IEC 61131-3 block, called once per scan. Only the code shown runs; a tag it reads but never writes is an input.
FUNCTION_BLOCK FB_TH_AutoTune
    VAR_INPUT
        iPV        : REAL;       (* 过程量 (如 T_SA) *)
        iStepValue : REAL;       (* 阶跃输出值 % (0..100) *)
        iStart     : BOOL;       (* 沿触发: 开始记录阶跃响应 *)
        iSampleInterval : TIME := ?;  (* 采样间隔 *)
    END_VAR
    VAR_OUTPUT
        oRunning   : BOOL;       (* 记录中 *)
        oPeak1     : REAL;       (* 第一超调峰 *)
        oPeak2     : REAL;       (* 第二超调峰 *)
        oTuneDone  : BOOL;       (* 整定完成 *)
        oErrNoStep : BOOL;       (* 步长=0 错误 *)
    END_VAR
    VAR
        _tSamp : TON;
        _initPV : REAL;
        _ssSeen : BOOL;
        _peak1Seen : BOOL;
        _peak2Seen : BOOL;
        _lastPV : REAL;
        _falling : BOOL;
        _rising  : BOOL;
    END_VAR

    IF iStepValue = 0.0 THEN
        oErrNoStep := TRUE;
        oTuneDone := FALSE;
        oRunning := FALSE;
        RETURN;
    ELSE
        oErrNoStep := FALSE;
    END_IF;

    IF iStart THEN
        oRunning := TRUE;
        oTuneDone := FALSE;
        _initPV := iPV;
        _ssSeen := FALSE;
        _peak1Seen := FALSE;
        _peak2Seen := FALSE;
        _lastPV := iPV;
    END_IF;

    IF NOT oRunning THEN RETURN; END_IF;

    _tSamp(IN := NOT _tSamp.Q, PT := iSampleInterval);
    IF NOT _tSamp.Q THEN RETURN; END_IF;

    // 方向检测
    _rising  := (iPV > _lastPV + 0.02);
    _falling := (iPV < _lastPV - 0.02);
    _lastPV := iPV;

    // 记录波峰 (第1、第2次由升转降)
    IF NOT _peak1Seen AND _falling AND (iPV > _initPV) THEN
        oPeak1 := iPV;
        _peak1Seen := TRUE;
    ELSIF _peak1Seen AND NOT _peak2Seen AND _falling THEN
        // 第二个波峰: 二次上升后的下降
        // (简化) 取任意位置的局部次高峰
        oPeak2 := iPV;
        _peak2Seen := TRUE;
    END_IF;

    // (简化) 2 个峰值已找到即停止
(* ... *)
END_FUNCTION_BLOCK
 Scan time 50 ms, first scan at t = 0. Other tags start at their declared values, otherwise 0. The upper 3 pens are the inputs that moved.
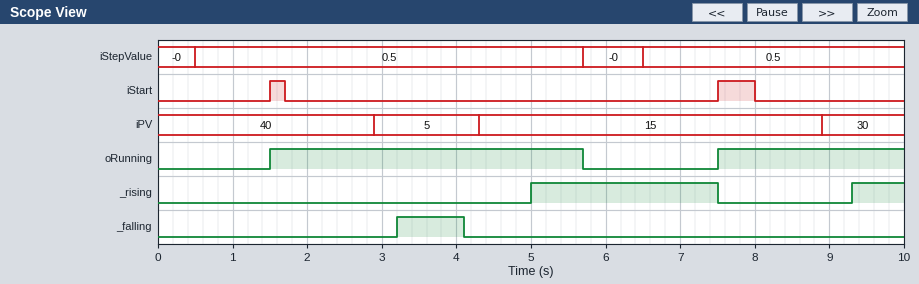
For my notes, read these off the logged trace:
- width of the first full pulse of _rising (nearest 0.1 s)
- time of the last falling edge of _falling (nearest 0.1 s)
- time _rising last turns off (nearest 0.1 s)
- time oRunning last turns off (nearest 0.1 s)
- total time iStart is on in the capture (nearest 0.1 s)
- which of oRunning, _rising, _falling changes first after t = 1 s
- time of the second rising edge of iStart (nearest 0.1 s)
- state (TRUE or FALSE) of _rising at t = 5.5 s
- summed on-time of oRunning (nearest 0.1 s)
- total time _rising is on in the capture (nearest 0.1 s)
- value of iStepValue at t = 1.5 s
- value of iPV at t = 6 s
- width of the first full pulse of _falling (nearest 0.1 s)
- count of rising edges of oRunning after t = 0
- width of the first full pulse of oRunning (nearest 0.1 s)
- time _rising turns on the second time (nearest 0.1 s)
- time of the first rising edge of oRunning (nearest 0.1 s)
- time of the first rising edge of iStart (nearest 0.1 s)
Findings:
2.5 s
4.1 s
7.5 s
5.7 s
0.7 s
oRunning
7.5 s
TRUE
6.7 s
3.2 s
0.5
15
0.9 s
2
4.2 s
9.3 s
1.5 s
1.5 s
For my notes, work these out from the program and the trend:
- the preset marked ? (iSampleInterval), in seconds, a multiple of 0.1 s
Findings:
0.8 s
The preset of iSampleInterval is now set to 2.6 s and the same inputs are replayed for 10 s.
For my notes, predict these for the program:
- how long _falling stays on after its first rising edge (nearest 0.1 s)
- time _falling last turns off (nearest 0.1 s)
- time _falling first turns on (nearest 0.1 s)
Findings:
3.4 s
7.5 s
4.1 s
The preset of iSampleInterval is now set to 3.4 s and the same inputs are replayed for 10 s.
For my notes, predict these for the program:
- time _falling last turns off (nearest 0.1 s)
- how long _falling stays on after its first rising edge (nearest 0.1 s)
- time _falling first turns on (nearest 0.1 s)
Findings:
8.4 s
3.5 s
4.9 s
